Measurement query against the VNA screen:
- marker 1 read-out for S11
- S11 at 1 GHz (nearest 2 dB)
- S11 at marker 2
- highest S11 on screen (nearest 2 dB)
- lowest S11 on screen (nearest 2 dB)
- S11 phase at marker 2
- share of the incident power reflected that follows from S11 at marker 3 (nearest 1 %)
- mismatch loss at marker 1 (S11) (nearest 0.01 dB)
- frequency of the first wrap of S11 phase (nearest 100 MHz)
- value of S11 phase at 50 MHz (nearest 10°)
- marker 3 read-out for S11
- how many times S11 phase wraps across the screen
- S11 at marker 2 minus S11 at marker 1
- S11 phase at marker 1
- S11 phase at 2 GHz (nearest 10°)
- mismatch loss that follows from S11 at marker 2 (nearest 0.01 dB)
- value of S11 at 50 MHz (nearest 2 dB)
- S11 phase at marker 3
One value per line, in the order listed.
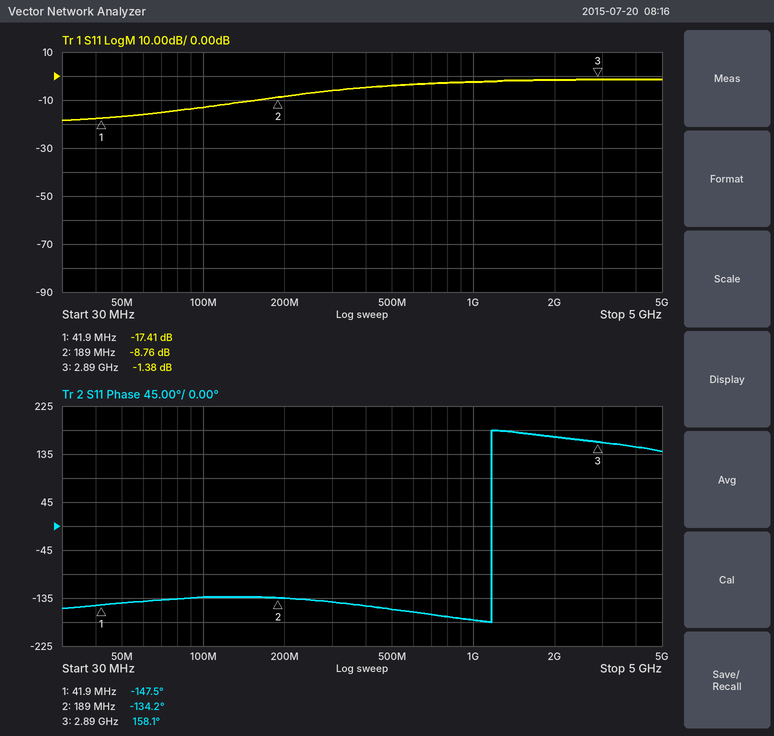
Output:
-17.41 dB
-2 dB
-8.76 dB
-2 dB
-18 dB
-134.2°
73 %
0.08 dB
1.2 GHz
-140°
-1.38 dB
1
8.65 dB
-147.5°
170°
0.62 dB
-16 dB
158.1°
